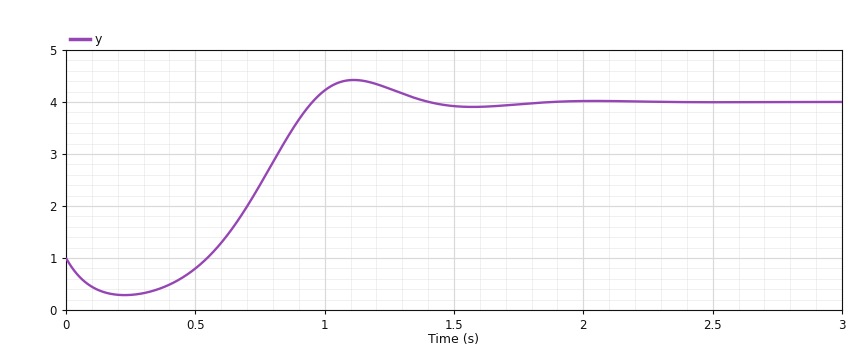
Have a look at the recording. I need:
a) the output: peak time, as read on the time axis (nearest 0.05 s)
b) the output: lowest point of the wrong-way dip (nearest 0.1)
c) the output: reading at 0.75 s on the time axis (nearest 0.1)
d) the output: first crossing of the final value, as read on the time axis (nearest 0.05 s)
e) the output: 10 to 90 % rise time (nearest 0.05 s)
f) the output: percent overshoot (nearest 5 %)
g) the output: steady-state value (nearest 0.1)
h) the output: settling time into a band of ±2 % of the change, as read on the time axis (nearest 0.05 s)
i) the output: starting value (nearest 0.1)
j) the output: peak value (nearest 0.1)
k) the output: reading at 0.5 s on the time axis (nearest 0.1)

1.10 s
0.3
2.4
0.95 s
0.30 s
15 %
4.0
1.70 s
1.0
4.4
0.8
